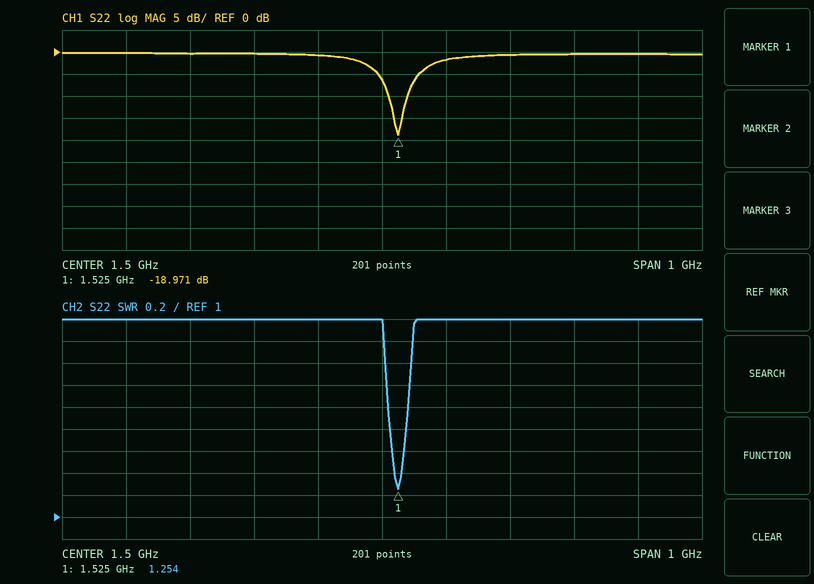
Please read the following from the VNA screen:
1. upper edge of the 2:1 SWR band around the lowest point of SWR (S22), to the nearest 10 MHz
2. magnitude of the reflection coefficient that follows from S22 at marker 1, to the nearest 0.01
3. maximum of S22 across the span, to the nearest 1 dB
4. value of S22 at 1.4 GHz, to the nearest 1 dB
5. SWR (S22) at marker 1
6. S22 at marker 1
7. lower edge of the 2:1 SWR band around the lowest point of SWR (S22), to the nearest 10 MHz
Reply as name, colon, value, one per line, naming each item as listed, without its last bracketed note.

upper edge of the 2:1 SWR band around the lowest point of SWR (S22), to the nearest 10 MHz: 1.54 GHz
magnitude of the reflection coefficient that follows from S22 at marker 1, to the nearest 0.01: 0.11
maximum of S22 across the span, to the nearest 1 dB: 0 dB
value of S22 at 1.4 GHz, to the nearest 1 dB: -1 dB
SWR (S22) at marker 1: 1.254
S22 at marker 1: -18.971 dB
lower edge of the 2:1 SWR band around the lowest point of SWR (S22), to the nearest 10 MHz: 1.51 GHz
